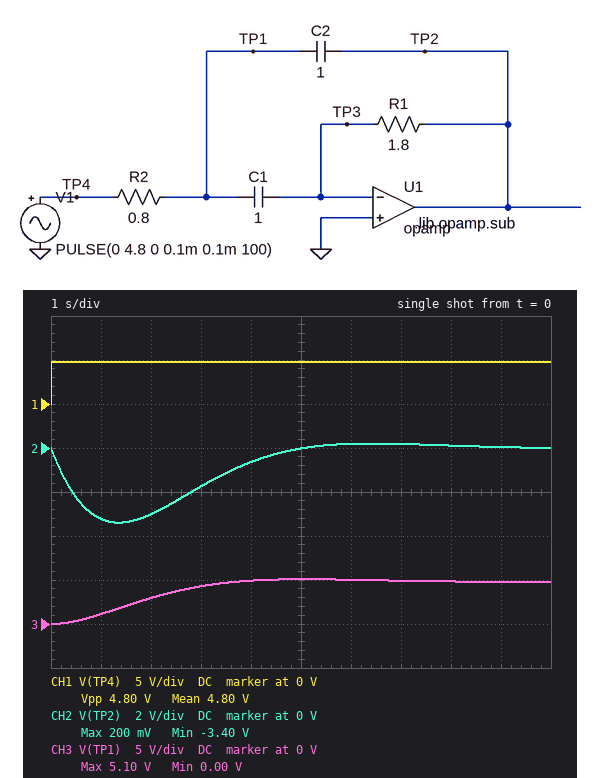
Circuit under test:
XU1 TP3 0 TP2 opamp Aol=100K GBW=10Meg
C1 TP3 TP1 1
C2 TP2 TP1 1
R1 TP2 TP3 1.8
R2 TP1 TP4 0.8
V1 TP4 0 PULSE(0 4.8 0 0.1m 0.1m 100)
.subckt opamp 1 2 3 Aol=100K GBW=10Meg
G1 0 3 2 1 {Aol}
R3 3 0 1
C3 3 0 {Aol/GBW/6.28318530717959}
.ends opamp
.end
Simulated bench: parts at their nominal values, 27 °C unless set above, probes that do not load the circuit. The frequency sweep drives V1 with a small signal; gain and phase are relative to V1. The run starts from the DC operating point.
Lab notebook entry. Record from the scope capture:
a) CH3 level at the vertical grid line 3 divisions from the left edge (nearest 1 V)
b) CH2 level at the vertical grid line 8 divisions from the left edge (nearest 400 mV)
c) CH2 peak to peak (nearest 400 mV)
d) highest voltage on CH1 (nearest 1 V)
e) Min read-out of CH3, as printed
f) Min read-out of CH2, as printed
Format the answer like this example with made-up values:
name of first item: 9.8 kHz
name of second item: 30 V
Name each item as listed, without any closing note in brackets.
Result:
CH3 level at the vertical grid line 3 divisions from the left edge: 4 V
CH2 level at the vertical grid line 8 divisions from the left edge: 0 V
CH2 peak to peak: 3.6 V
highest voltage on CH1: 5 V
Min read-out of CH3, as printed: 0.00 V
Min read-out of CH2, as printed: -3.40 V
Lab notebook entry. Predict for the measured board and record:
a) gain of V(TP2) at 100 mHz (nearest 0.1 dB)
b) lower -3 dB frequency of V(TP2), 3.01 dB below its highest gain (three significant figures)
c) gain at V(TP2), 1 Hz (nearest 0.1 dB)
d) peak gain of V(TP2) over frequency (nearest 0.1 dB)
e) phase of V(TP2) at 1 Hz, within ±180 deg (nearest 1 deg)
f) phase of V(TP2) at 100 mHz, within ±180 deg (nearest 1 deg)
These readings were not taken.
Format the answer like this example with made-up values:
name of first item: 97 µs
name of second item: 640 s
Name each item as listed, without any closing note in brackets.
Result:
gain of V(TP2) at 100 mHz: 0.3 dB
lower -3 dB frequency of V(TP2), 3.01 dB below its highest gain: 71.0 mHz
gain at V(TP2), 1 Hz: -14.0 dB
peak gain of V(TP2) over frequency: 1.0 dB
phase of V(TP2) at 1 Hz, within ±180 deg: 100 deg
phase of V(TP2) at 100 mHz, within ±180 deg: -157 deg
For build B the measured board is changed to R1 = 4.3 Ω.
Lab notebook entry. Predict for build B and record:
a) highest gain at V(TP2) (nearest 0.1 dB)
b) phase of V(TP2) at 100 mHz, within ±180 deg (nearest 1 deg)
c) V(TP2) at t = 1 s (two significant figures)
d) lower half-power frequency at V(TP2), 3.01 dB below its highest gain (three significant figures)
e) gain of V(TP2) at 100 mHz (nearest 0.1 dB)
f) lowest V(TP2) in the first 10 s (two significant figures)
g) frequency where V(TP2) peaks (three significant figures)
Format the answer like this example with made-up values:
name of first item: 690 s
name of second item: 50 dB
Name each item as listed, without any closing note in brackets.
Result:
highest gain at V(TP2): 8.6 dB
phase of V(TP2) at 100 mHz, within ±180 deg: 160 deg
V(TP2) at t = 1 s: -4.6 V
lower half-power frequency at V(TP2), 3.01 dB below its highest gain: 56.4 mHz
gain of V(TP2) at 100 mHz: 8.1 dB
lowest V(TP2) in the first 10 s: -6.5 V
frequency where V(TP2) peaks: 85.8 mHz
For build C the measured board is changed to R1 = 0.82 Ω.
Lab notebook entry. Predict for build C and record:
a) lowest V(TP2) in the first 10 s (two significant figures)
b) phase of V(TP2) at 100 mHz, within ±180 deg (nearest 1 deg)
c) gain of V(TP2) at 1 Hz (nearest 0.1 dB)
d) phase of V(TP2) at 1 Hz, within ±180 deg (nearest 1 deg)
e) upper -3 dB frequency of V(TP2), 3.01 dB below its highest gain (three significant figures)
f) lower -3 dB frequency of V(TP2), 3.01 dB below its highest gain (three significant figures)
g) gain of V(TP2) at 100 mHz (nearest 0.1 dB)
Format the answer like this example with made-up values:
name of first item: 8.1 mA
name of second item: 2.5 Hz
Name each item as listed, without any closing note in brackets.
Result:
lowest V(TP2) in the first 10 s: -1.8 V
phase of V(TP2) at 100 mHz, within ±180 deg: -144 deg
gain of V(TP2) at 1 Hz: -14.3 dB
phase of V(TP2) at 1 Hz, within ±180 deg: 112 deg
upper -3 dB frequency of V(TP2), 3.01 dB below its highest gain: 470 mHz
lower -3 dB frequency of V(TP2), 3.01 dB below its highest gain: 82.1 mHz
gain of V(TP2) at 100 mHz: -7.7 dB
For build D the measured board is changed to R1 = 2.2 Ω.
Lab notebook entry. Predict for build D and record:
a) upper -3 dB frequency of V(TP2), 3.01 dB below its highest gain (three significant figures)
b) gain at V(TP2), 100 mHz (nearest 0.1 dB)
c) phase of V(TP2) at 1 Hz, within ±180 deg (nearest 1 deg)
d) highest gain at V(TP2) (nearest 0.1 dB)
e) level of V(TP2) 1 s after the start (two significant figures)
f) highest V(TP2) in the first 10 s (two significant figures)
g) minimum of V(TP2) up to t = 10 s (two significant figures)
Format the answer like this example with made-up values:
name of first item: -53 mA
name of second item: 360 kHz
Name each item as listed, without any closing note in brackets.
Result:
upper -3 dB frequency of V(TP2), 3.01 dB below its highest gain: 212 mHz
gain at V(TP2), 100 mHz: 2.4 dB
phase of V(TP2) at 1 Hz, within ±180 deg: 98 deg
highest gain at V(TP2): 2.8 dB
level of V(TP2) 1 s after the start: -3.6 V
highest V(TP2) in the first 10 s: 370 mV
minimum of V(TP2) up to t = 10 s: -4.0 V
